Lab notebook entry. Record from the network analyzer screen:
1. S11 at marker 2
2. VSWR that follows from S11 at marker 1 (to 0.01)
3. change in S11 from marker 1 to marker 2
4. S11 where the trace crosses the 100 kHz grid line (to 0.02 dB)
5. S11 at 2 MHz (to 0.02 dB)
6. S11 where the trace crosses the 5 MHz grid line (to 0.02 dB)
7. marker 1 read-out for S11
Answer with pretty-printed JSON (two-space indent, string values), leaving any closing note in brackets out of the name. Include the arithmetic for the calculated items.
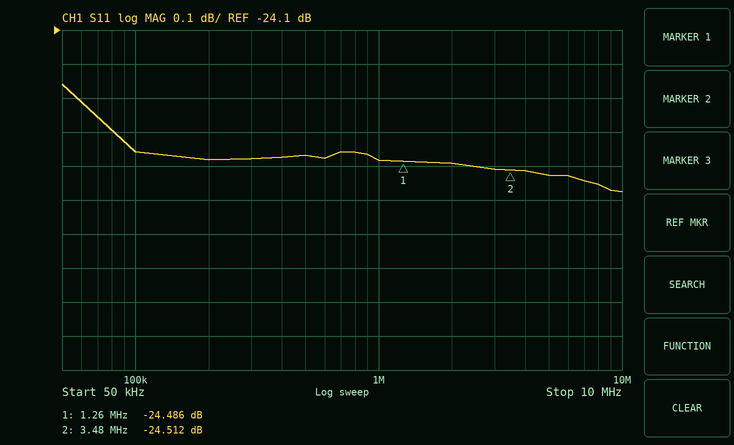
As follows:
{
  "S11 at marker 2": "-24.512 dB",
  "VSWR that follows from S11 at marker 1": "(1 + 0.0597)/(1 − 0.0597) ≈ 1.13",
  "change in S11 from marker 1 to marker 2": "-24.512 − (-24.486) = -0.026 dB",
  "S11 where the trace crosses the 100 kHz grid line": "-24.46 dB",
  "S11 at 2 MHz": "-24.50 dB",
  "S11 where the trace crosses the 5 MHz grid line": "-24.52 dB",
  "marker 1 read-out for S11": "-24.486 dB"
}
